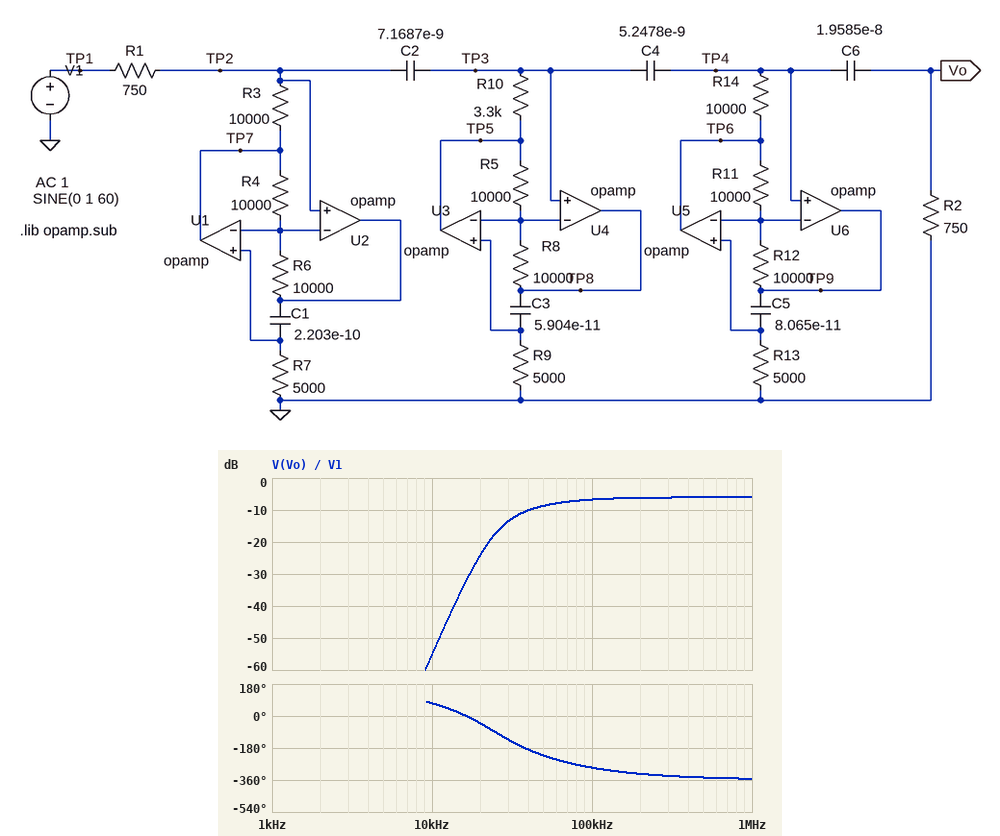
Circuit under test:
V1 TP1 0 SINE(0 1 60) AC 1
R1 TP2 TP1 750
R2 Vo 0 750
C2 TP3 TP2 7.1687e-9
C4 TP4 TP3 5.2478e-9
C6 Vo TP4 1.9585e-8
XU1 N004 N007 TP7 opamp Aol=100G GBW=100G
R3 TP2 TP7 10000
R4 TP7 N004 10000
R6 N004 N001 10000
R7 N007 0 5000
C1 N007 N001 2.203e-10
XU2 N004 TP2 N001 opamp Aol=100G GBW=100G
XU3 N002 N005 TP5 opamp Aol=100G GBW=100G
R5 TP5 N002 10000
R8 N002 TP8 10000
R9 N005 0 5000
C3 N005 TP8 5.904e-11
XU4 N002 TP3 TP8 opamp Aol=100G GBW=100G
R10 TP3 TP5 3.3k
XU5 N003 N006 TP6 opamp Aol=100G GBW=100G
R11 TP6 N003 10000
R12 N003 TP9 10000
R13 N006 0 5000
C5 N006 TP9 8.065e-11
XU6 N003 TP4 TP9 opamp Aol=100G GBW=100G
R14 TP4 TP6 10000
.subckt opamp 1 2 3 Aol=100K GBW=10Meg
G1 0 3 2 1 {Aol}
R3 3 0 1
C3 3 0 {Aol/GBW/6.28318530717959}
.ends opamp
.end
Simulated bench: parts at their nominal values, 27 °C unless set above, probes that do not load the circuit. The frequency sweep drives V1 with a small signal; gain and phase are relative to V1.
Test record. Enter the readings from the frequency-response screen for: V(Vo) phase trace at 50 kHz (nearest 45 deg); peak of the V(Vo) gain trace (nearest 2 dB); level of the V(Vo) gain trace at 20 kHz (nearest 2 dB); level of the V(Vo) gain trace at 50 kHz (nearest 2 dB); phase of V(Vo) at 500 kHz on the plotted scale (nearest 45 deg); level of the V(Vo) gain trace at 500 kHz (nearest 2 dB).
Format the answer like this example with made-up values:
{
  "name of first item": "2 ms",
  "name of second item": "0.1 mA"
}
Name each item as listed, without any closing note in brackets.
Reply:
{
  "V(Vo) phase trace at 50 kHz": "-225 deg",
  "peak of the V(Vo) gain trace": "-6 dB",
  "level of the V(Vo) gain trace at 20 kHz": "-24 dB",
  "level of the V(Vo) gain trace at 50 kHz": "-8 dB",
  "phase of V(Vo) at 500 kHz on the plotted scale": "-360 deg",
  "level of the V(Vo) gain trace at 500 kHz": "-6 dB"
}
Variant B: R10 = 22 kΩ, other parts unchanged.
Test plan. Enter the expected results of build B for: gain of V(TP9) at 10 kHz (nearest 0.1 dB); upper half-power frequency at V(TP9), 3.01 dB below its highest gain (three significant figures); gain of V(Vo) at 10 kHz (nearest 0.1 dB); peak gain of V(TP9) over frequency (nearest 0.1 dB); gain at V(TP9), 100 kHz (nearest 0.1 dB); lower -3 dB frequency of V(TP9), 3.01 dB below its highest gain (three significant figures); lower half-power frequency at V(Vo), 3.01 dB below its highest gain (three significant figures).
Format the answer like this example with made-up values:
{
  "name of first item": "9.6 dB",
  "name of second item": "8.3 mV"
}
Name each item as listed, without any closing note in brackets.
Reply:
{
  "gain of V(TP9) at 10 kHz": "0 dB",
  "upper half-power frequency at V(TP9), 3.01 dB below its highest gain": "21.8 kHz",
  "gain of V(Vo) at 10 kHz": "-35.3 dB",
  "peak gain of V(TP9) over frequency": "21.5 dB",
  "gain at V(TP9), 100 kHz": "6.2 dB",
  "lower -3 dB frequency of V(TP9), 3.01 dB below its highest gain": "14.4 kHz",
  "lower half-power frequency at V(Vo), 3.01 dB below its highest gain": "15.4 kHz"
}
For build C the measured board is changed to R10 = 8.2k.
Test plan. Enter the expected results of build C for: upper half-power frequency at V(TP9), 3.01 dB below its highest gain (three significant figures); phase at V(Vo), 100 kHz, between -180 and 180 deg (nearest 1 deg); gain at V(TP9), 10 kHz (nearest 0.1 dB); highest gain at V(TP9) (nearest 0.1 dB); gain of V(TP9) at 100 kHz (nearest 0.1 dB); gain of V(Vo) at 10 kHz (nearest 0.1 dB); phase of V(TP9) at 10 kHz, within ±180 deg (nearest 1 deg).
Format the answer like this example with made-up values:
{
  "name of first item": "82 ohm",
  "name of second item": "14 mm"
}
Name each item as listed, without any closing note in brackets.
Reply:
{
  "upper half-power frequency at V(TP9), 3.01 dB below its highest gain": "40.0 kHz",
  "phase at V(Vo), 100 kHz, between -180 and 180 deg": "49 deg",
  "gain at V(TP9), 10 kHz": "-11.2 dB",
  "highest gain at V(TP9)": "17.1 dB",
  "gain of V(TP9) at 100 kHz": "6.2 dB",
  "gain of V(Vo) at 10 kHz": "-46.5 dB",
  "phase of V(TP9) at 10 kHz, within ±180 deg": "-65 deg"
}
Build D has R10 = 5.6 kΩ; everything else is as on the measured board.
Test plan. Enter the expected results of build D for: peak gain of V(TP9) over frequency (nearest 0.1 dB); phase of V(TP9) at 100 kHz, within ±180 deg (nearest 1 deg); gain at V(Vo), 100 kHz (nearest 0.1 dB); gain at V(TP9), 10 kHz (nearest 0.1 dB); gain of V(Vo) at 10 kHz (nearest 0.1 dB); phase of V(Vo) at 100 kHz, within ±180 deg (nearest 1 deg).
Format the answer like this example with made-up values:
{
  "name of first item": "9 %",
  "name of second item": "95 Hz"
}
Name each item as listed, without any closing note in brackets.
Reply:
{
  "peak gain of V(TP9) over frequency": "14.4 dB",
  "phase of V(TP9) at 100 kHz, within ±180 deg": "-26 deg",
  "gain at V(Vo), 100 kHz": "-6.1 dB",
  "gain at V(TP9), 10 kHz": "-15.0 dB",
  "gain of V(Vo) at 10 kHz": "-50.3 dB",
  "phase of V(Vo) at 100 kHz, within ±180 deg": "56 deg"
}
